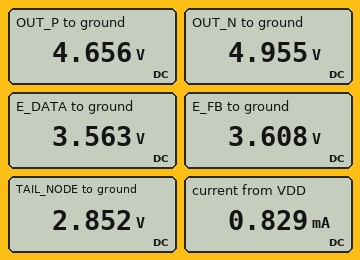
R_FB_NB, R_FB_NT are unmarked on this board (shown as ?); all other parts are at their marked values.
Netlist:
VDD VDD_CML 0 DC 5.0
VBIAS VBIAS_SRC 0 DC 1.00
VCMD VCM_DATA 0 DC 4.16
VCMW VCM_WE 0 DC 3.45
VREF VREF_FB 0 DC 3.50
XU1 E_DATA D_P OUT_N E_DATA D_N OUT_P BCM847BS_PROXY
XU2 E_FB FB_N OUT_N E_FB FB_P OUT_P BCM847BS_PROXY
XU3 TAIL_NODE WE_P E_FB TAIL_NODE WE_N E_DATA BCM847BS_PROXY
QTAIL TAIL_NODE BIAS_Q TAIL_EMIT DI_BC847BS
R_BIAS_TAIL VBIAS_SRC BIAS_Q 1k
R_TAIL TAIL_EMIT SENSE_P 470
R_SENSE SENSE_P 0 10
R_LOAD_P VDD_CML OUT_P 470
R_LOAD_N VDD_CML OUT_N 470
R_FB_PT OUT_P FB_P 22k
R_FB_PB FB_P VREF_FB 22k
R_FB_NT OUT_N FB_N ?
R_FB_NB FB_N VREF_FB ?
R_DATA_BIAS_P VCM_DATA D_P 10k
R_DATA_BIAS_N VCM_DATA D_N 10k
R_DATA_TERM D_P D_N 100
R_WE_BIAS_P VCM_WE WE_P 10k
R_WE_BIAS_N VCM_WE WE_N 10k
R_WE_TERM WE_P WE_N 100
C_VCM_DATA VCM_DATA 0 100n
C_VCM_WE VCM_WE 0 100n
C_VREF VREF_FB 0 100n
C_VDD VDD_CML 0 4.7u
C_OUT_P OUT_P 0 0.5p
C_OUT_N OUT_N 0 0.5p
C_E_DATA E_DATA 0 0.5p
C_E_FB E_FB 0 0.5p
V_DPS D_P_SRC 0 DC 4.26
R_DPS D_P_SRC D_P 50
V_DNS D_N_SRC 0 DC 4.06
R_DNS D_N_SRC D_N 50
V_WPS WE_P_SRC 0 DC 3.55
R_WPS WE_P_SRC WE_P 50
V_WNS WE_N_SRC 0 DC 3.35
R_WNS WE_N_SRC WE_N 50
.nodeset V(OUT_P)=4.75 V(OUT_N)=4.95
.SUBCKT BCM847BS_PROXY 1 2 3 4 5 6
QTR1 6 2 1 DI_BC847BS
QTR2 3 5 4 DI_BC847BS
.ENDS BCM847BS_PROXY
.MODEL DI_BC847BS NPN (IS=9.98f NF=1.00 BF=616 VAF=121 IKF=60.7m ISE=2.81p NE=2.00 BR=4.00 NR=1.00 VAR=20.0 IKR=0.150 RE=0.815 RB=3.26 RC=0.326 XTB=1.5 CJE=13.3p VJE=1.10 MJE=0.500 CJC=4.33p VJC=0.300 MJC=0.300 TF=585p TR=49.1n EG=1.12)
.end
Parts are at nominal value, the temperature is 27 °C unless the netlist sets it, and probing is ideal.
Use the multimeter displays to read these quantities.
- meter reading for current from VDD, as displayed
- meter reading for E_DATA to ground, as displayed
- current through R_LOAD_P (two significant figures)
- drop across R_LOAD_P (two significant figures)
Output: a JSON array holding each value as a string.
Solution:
["0.829 mA", "3.563 V", "730 µA", "340 mV"]
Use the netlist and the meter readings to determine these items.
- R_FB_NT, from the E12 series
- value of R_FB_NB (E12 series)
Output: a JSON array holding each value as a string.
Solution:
["10 kΩ", "8.2 kΩ"]
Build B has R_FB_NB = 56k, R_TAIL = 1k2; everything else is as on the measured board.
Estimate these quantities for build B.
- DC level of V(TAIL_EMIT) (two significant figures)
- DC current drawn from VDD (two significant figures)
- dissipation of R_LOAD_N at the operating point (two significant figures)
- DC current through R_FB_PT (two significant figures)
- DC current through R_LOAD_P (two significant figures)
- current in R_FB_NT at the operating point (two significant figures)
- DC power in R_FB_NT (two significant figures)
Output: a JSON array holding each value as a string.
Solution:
["370 mV", "360 µA", "390 nW", "31 µA", "330 µA", "23 µA", "5.1 µW"]
